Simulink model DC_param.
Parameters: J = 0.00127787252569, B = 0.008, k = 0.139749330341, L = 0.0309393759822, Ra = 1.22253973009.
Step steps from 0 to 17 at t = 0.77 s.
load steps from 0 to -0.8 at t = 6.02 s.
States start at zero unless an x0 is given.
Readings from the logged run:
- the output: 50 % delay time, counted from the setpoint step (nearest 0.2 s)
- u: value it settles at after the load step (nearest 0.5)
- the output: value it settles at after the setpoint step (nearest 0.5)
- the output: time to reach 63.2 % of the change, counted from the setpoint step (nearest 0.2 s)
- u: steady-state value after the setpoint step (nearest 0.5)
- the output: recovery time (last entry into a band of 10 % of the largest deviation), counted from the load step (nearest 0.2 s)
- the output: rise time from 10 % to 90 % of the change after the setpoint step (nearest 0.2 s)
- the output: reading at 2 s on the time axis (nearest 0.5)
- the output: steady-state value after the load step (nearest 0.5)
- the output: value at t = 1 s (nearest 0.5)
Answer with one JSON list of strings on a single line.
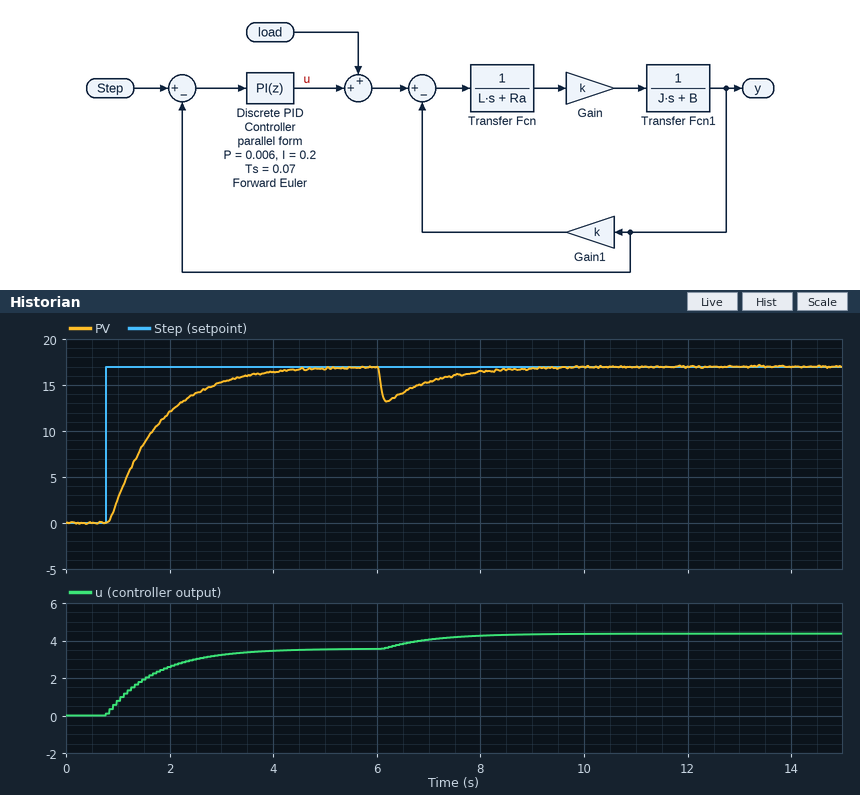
["0.8 s", "4.5", "17.0", "1.0 s", "3.5", "2.4 s", "2.0 s", "12.0", "17.0", "2.5"]
